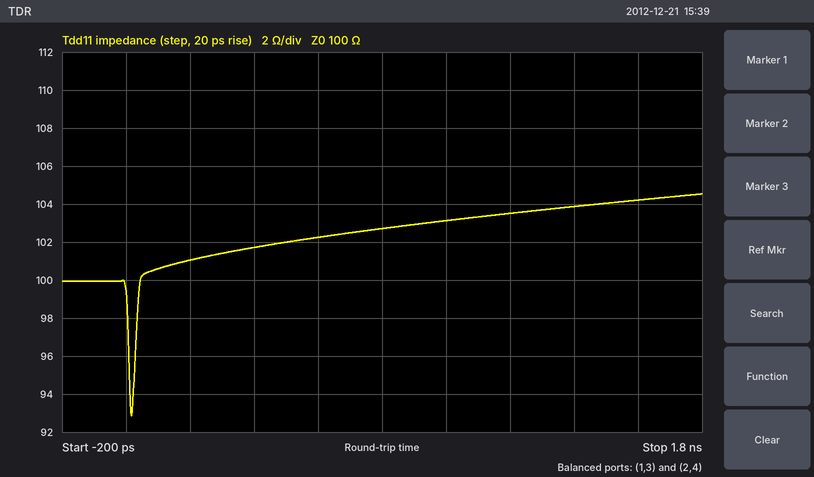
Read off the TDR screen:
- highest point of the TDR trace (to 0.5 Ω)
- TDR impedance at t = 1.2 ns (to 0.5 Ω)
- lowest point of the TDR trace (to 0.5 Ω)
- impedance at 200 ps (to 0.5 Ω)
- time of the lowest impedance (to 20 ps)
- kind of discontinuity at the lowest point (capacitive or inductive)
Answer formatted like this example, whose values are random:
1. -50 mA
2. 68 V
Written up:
1. 104.5 Ω
2. 103.5 Ω
3. 93.0 Ω
4. 101.0 Ω
5. 20 ps
6. capacitive
